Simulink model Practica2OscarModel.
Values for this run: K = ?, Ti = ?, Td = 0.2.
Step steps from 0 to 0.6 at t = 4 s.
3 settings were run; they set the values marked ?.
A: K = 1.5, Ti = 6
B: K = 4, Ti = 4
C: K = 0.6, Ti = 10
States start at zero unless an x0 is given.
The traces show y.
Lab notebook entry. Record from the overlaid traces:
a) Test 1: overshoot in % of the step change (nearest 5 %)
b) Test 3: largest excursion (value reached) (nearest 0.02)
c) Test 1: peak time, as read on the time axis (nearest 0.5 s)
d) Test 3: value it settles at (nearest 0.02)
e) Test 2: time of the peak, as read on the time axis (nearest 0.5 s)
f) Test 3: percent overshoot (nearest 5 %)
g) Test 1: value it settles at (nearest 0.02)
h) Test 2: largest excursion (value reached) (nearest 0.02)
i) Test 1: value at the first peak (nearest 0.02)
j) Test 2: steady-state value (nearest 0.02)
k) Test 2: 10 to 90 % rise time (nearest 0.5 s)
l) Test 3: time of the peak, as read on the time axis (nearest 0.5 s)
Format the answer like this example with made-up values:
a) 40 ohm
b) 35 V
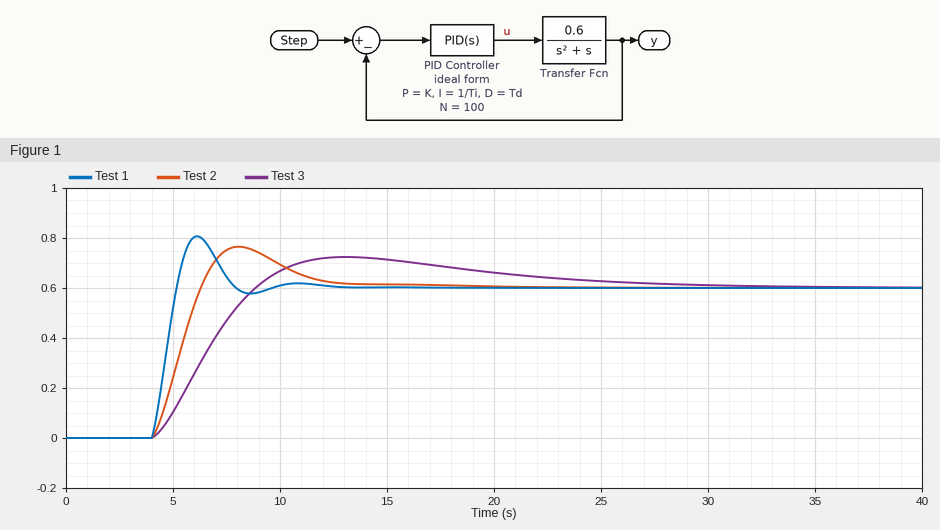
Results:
a) 35 %
b) 0.72
c) 6.0 s
d) 0.60
e) 8.0 s
f) 20 %
g) 0.60
h) 0.76
i) 0.80
j) 0.60
k) 1.5 s
l) 13.0 s
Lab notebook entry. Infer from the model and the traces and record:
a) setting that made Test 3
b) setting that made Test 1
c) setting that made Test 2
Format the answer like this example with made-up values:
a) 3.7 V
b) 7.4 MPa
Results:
a) C
b) B
c) A
